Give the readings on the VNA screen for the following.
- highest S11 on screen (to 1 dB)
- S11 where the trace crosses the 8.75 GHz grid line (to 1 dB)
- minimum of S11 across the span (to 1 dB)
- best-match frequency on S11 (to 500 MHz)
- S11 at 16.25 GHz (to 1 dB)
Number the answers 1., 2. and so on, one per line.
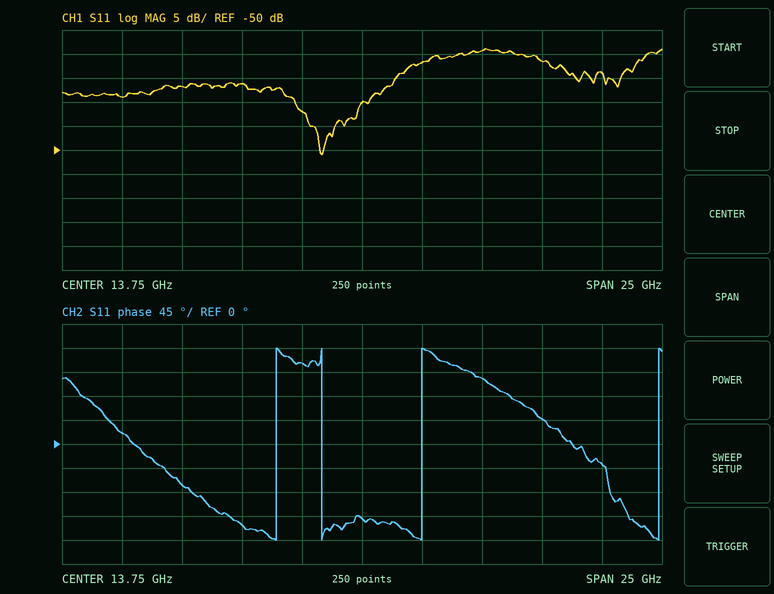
1. -29 dB
2. -36 dB
3. -51 dB
4. 12.0 GHz
5. -32 dB
